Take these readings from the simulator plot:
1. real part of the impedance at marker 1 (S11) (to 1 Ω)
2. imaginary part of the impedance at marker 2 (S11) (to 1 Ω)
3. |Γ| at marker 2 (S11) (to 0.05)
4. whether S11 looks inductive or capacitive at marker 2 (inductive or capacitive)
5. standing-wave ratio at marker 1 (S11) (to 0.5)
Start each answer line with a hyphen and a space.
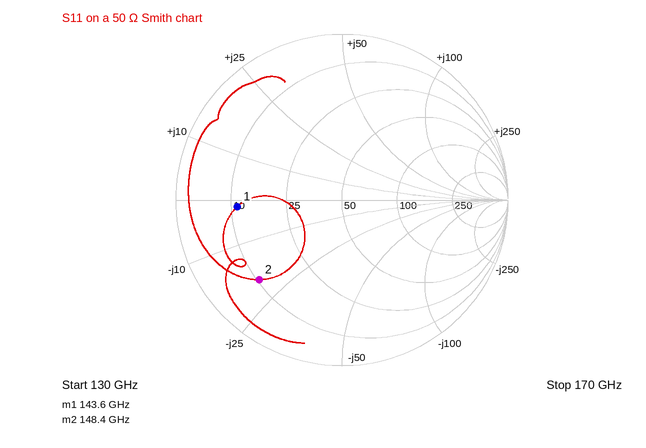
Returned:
- 11 Ω
- -19 Ω
- 0.70
- capacitive
- 4.5
